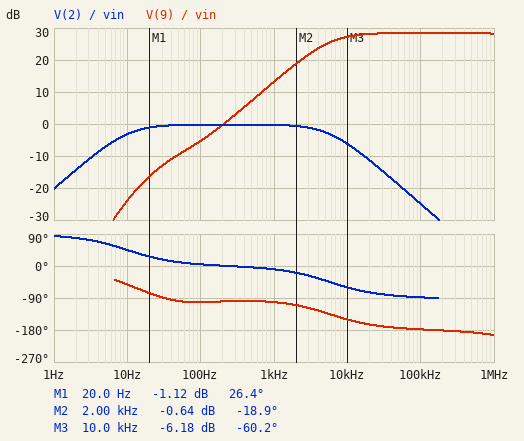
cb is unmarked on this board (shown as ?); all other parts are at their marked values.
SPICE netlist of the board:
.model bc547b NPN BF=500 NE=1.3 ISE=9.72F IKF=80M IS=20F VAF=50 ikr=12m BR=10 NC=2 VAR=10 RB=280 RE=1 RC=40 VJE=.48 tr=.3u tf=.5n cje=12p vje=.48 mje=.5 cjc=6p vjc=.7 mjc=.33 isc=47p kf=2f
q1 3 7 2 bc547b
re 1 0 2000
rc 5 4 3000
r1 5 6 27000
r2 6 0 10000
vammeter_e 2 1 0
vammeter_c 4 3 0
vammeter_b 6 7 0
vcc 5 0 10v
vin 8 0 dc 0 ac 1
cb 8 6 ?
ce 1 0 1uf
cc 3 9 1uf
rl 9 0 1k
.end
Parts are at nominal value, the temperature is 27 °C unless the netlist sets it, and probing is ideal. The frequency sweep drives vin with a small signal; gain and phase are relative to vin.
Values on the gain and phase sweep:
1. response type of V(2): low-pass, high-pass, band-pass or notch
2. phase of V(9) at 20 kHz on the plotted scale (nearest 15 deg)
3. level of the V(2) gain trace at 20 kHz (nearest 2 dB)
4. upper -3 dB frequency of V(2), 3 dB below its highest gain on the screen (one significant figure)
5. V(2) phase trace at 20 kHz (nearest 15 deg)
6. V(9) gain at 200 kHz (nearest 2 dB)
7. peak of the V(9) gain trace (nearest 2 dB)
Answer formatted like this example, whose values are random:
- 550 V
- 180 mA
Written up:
- band-pass
- -165 deg
- -12 dB
- 6 kHz
- -75 deg
- 28 dB
- 28 dB
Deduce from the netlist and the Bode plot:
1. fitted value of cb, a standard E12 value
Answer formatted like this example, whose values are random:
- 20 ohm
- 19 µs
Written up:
- 2.2 µF
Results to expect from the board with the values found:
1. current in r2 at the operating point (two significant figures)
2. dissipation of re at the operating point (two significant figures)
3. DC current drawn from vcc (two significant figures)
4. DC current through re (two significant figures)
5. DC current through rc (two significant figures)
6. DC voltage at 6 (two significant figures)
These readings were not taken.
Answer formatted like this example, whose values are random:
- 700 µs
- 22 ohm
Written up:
- 270 µA
- 2.1 mW
- 1.3 mA
- 1.0 mA
- 1.0 mA
- 2.7 V
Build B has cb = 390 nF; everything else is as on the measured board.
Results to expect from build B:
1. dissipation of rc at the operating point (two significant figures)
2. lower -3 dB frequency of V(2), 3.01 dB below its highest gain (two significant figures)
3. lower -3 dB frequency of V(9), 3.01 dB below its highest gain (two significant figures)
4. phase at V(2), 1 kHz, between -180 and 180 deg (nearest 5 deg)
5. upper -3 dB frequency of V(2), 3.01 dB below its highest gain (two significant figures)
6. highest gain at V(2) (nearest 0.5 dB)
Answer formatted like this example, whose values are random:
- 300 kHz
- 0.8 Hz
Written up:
- 3.1 mW
- 55 Hz
- 5.8 kHz
- -5 deg
- 5.9 kHz
- -0.5 dB
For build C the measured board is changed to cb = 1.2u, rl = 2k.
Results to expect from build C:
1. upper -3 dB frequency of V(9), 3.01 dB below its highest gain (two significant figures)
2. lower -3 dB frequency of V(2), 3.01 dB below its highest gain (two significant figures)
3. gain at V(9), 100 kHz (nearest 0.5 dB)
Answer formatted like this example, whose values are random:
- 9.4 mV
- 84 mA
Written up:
- 2.9 MHz
- 18 Hz
- 32.5 dB
